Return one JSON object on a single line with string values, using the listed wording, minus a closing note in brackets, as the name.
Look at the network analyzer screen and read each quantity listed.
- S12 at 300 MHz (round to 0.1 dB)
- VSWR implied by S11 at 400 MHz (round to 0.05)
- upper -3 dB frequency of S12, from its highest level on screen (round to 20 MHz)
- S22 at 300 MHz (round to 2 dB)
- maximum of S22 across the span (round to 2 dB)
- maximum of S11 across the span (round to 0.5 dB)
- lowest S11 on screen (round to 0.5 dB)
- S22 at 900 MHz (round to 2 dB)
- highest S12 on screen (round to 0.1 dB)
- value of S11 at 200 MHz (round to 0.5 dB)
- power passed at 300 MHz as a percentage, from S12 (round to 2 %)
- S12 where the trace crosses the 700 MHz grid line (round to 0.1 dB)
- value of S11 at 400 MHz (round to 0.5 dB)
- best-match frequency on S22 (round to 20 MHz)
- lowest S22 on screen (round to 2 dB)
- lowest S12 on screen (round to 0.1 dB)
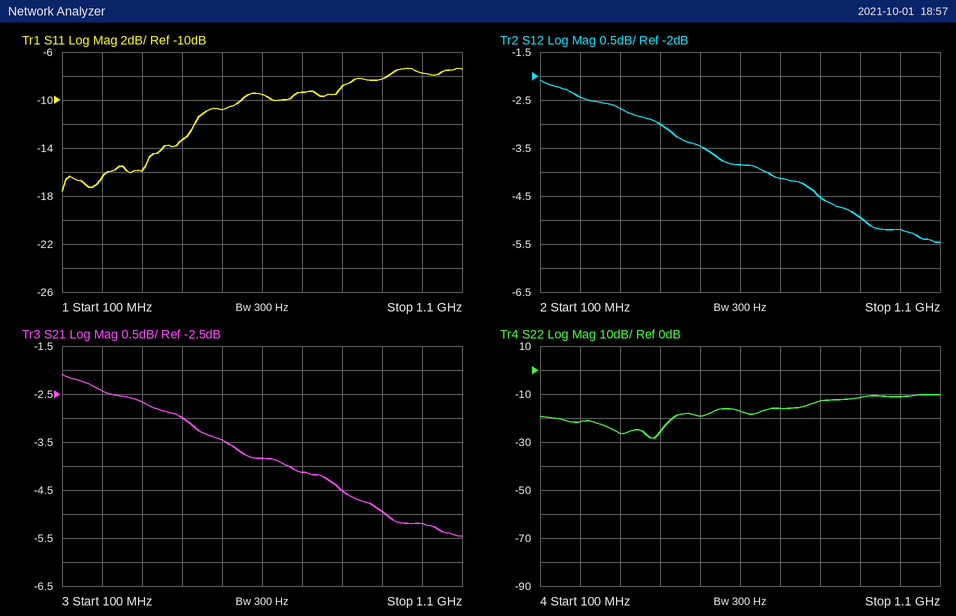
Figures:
{"S12 at 300 MHz": "-2.7 dB", "VSWR implied by S11 at 400 MHz": "1.55", "upper -3 dB frequency of S12, from its highest level on screen": "920 MHz", "S22 at 300 MHz": "-26 dB", "maximum of S22 across the span": "-10 dB", "maximum of S11 across the span": "-7.5 dB", "lowest S11 on screen": "-17.5 dB", "S22 at 900 MHz": "-12 dB", "highest S12 on screen": "-2.1 dB", "value of S11 at 200 MHz": "-16.5 dB", "power passed at 300 MHz as a percentage, from S12": "54 %", "S12 where the trace crosses the 700 MHz grid line": "-4.1 dB", "value of S11 at 400 MHz": "-13.5 dB", "best-match frequency on S22": "380 MHz", "lowest S22 on screen": "-28 dB", "lowest S12 on screen": "-5.5 dB"}
